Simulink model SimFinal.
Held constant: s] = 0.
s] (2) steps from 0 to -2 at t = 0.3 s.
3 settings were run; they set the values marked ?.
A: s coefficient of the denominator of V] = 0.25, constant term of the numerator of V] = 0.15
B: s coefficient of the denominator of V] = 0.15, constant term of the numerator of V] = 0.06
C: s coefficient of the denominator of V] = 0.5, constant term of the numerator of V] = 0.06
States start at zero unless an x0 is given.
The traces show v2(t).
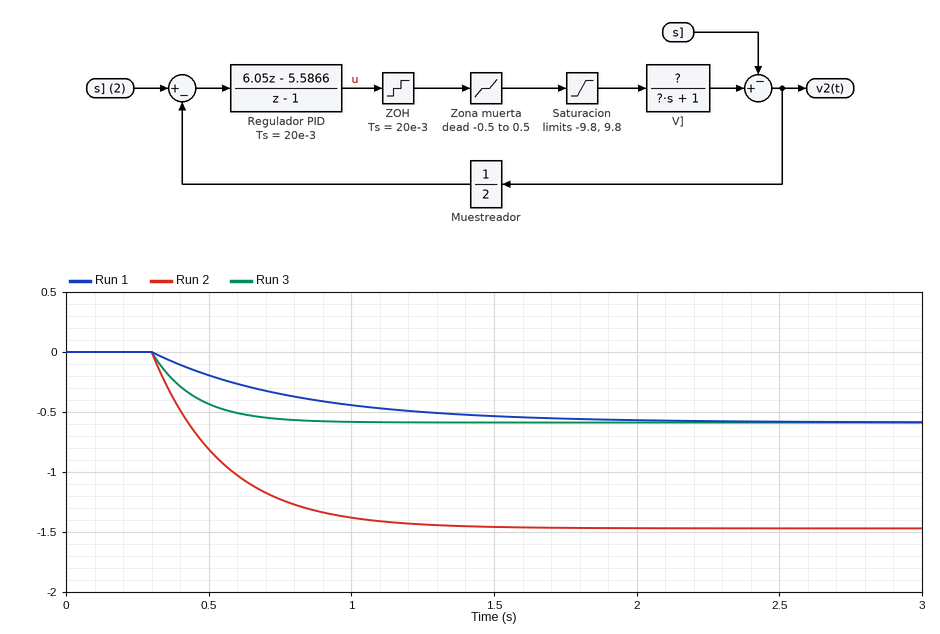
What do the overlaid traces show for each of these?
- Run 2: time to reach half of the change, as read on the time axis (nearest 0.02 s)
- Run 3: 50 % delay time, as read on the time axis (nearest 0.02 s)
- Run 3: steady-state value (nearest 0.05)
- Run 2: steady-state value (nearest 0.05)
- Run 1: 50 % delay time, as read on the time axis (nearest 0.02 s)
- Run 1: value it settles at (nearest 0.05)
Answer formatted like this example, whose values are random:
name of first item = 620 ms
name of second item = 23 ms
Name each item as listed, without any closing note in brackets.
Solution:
Run 2: time to reach half of the change, as read on the time axis = 0.48 s
Run 3: 50 % delay time, as read on the time axis = 0.40 s
Run 3: steady-state value = -0.60
Run 2: steady-state value = -1.45
Run 1: 50 % delay time, as read on the time axis = 0.64 s
Run 1: value it settles at = -0.60
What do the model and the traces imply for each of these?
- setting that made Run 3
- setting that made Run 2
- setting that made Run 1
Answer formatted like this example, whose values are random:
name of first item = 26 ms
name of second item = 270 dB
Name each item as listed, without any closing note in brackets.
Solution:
setting that made Run 3 = B
setting that made Run 2 = A
setting that made Run 1 = C
